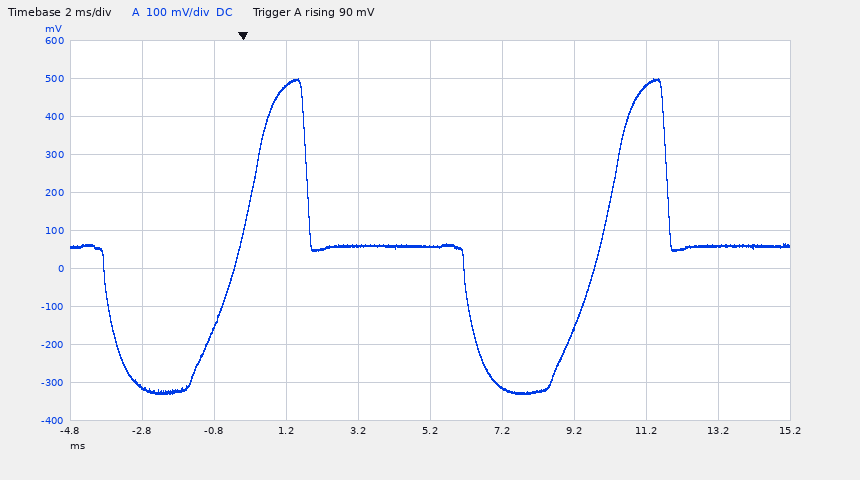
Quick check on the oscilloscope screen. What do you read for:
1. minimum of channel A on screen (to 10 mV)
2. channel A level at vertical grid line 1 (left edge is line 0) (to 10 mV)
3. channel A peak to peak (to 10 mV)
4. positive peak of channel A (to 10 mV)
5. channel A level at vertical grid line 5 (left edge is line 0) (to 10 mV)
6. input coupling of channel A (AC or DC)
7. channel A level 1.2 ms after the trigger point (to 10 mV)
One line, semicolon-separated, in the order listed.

-330 mV; -310 mV; 830 mV; 500 mV; 60 mV; DC; 480 mV
